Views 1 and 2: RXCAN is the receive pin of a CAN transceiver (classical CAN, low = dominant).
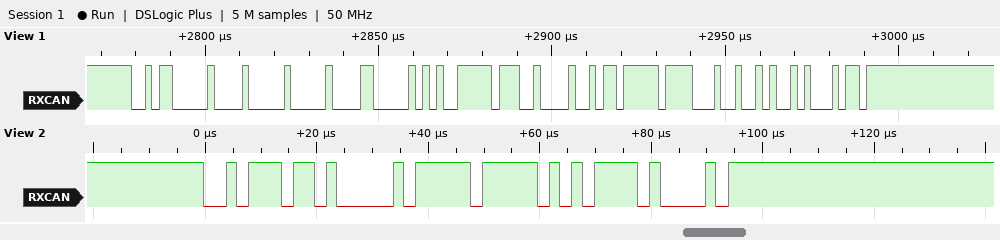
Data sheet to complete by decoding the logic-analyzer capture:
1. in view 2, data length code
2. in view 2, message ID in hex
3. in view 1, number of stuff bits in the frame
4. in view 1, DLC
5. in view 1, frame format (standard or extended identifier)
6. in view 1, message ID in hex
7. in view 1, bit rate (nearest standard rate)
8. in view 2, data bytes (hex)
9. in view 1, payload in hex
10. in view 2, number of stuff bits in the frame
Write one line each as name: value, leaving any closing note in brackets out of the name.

in view 2, data length code: 1
in view 2, message ID in hex: 0x2ED
in view 1, number of stuff bits in the frame: 6
in view 1, DLC: 8
in view 1, frame format: standard
in view 1, message ID in hex: 0x2C0
in view 1, bit rate: 500 kbit/s
in view 2, data bytes: FF
in view 1, payload in hex: 00 18 14 FF 21 2D FF 12
in view 2, number of stuff bits in the frame: 3
